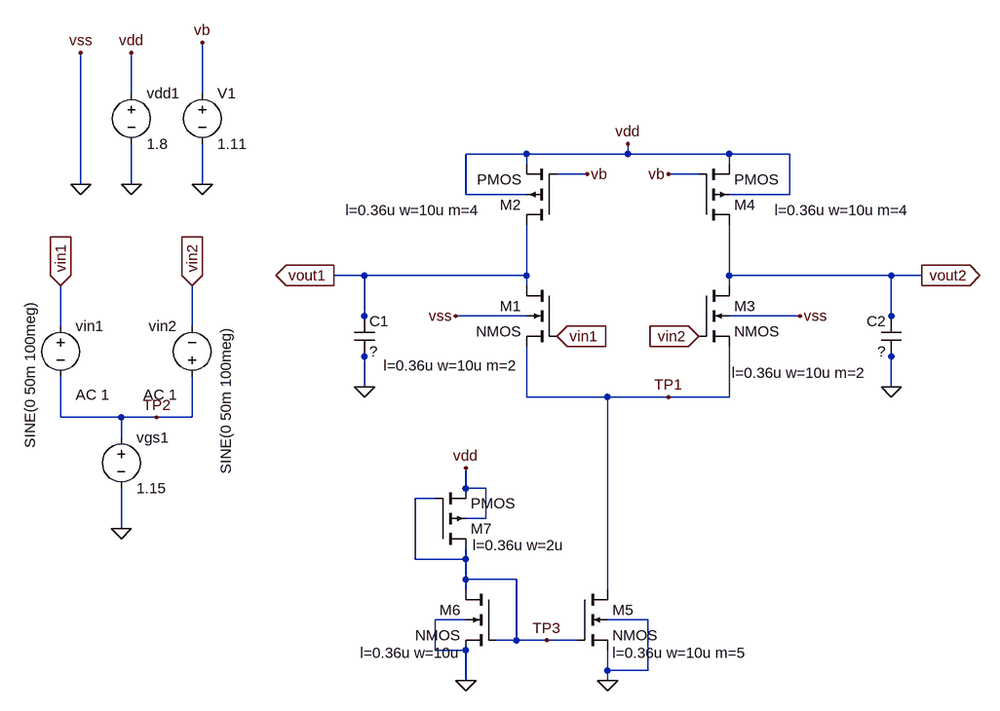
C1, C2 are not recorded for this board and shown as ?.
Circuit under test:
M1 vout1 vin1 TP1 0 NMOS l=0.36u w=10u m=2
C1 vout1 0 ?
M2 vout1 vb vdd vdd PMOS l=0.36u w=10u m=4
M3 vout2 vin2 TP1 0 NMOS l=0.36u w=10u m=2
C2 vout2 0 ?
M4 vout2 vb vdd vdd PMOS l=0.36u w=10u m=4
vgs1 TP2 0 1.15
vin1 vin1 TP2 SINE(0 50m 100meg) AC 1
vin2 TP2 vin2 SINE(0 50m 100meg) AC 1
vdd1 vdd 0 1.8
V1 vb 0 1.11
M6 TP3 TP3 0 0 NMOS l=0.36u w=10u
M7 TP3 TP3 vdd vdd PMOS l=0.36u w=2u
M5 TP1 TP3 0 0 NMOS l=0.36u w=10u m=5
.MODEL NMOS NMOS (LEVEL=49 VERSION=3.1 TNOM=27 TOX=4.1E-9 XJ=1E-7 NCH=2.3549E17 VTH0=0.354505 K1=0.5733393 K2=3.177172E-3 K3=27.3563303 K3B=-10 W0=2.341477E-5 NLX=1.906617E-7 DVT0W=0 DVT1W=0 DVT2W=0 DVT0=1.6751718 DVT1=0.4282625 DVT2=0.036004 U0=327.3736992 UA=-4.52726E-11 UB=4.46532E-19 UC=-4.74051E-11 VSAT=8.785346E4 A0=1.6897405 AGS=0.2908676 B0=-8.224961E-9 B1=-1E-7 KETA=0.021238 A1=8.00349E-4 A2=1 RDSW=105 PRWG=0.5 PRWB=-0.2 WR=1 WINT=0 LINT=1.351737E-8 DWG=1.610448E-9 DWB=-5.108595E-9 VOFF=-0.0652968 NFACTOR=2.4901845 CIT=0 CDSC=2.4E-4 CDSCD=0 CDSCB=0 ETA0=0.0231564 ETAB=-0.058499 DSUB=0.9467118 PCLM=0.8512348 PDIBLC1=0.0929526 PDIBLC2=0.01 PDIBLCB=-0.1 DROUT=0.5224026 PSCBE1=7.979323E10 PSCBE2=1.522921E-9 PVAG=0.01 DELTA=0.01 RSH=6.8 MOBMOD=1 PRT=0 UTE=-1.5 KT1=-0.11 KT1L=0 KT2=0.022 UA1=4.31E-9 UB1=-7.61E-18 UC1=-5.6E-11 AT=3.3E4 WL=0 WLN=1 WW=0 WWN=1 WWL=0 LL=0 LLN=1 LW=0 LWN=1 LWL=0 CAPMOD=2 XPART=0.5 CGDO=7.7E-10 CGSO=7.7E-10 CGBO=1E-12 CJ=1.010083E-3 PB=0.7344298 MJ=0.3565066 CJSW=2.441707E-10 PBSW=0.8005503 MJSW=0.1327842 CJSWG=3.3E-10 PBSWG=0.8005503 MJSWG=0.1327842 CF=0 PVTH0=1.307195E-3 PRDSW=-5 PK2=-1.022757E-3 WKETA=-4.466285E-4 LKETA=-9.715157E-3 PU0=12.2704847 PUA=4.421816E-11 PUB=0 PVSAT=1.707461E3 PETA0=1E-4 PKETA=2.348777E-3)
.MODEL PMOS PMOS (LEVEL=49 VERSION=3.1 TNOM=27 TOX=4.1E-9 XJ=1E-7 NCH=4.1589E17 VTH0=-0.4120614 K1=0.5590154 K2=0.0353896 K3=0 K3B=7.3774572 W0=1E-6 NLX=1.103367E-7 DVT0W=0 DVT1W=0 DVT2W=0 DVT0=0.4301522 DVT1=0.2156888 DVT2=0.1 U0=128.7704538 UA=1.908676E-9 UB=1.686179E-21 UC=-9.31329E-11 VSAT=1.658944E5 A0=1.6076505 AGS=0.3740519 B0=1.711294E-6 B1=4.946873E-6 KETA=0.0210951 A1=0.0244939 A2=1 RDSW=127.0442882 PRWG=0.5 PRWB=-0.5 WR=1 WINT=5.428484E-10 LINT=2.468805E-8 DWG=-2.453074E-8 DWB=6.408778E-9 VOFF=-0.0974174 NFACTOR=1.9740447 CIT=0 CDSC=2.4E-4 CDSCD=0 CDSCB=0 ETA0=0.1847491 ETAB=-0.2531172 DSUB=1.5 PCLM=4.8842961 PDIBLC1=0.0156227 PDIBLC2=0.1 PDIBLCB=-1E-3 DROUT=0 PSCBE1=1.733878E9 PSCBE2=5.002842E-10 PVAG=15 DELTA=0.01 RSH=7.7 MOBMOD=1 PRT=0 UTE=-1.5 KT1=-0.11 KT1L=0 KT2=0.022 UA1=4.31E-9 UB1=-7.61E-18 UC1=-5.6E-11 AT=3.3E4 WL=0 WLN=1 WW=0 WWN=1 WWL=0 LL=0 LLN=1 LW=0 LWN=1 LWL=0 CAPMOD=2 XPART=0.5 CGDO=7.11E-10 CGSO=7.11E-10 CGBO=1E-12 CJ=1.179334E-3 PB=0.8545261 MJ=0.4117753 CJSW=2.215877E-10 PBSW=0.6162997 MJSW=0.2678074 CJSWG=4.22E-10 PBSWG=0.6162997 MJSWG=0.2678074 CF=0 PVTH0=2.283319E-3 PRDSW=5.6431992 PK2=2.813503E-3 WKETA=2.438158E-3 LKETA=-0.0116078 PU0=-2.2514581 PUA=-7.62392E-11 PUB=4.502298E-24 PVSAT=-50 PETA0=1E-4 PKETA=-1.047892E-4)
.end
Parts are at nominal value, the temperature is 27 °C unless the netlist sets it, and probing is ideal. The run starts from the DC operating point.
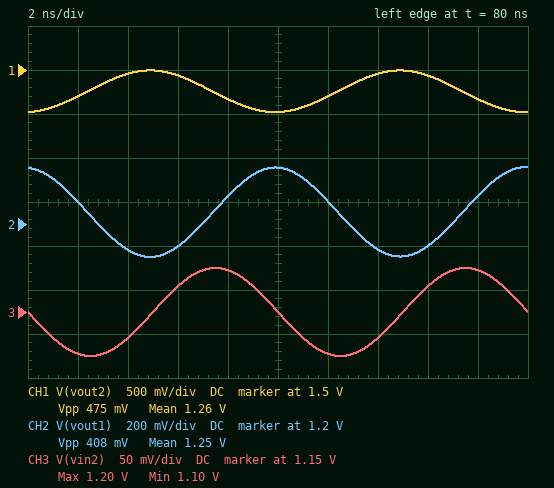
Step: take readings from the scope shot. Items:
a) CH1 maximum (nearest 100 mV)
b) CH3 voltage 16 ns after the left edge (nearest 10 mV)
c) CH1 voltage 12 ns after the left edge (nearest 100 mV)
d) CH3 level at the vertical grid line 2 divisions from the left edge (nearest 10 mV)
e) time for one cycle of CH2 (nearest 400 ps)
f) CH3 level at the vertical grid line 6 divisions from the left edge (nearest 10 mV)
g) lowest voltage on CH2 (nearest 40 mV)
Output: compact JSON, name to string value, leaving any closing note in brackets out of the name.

{"CH1 maximum": "1.5 V", "CH3 voltage 16 ns after the left edge": "1.18 V", "CH1 voltage 12 ns after the left edge": "1.2 V", "CH3 level at the vertical grid line 2 divisions from the left edge": "1.12 V", "time for one cycle of CH2": "10.0 ns", "CH3 level at the vertical grid line 6 divisions from the left edge": "1.10 V", "lowest voltage on CH2": "1.04 V"}
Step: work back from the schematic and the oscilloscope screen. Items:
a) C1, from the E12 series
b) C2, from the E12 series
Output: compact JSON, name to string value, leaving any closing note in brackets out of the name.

{"C1, from the E12 series": "820 fF", "C2, from the E12 series": "680 fF"}
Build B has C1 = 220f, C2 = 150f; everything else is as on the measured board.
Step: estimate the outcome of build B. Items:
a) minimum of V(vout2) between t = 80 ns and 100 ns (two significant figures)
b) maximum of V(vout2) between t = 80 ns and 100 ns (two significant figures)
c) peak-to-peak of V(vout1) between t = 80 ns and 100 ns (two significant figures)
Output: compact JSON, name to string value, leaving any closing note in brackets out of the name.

{"minimum of V(vout2) between t = 80 ns and 100 ns": "460 mV", "maximum of V(vout2) between t = 80 ns and 100 ns": "1.7 V", "peak-to-peak of V(vout1) between t = 80 ns and 100 ns": "1.1 V"}
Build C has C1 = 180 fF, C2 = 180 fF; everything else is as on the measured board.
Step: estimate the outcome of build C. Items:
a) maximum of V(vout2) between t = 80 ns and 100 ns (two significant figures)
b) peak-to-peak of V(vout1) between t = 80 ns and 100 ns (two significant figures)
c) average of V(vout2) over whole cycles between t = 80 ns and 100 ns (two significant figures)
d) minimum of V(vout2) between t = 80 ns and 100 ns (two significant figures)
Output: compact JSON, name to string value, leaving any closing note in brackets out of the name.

{"maximum of V(vout2) between t = 80 ns and 100 ns": "1.7 V", "peak-to-peak of V(vout1) between t = 80 ns and 100 ns": "1.2 V", "average of V(vout2) over whole cycles between t = 80 ns and 100 ns": "1.1 V", "minimum of V(vout2) between t = 80 ns and 100 ns": "480 mV"}
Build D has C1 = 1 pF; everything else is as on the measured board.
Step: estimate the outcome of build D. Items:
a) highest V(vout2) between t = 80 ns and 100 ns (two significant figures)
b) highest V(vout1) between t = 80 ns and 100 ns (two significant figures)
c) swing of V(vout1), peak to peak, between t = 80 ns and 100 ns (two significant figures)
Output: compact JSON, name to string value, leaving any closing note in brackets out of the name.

{"highest V(vout2) between t = 80 ns and 100 ns": "1.5 V", "highest V(vout1) between t = 80 ns and 100 ns": "1.4 V", "swing of V(vout1), peak to peak, between t = 80 ns and 100 ns": "340 mV"}
